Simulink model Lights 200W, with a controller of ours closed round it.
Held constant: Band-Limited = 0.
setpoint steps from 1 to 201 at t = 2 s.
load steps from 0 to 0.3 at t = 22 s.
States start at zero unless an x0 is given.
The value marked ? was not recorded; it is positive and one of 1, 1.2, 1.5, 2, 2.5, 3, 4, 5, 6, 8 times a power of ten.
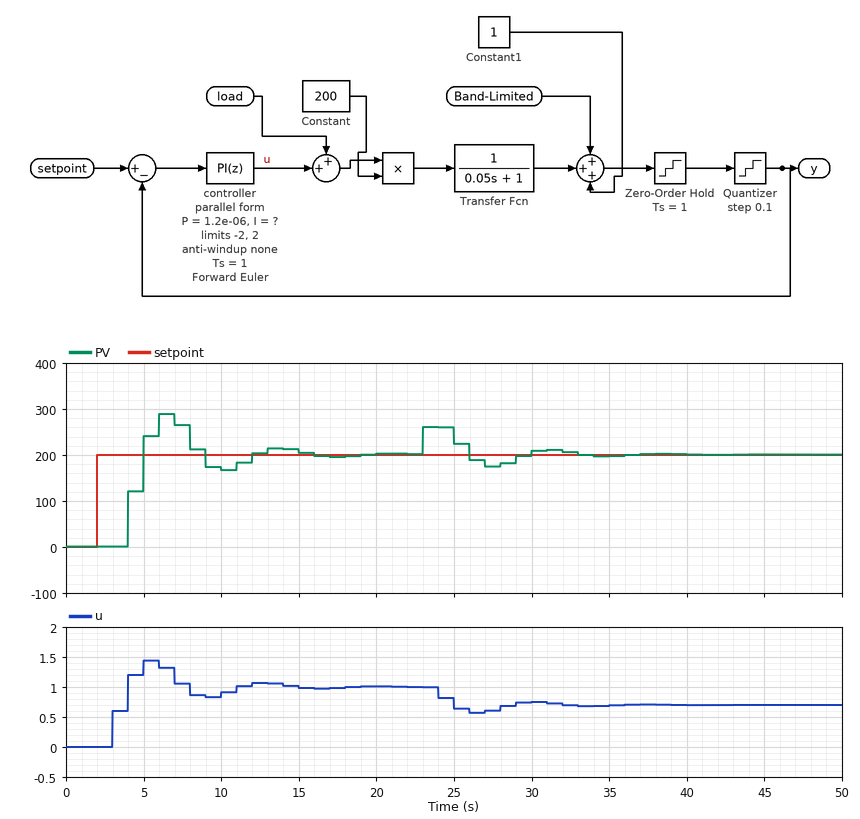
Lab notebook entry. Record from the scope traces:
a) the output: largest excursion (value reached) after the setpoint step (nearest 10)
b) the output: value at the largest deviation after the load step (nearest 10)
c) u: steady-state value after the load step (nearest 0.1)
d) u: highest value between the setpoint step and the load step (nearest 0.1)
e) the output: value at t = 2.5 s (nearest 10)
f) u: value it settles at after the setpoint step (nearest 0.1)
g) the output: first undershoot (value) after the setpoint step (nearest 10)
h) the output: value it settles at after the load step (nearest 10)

290
260
0.7
1.4
0
1.0
170
200
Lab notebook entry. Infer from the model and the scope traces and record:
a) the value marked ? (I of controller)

0.003
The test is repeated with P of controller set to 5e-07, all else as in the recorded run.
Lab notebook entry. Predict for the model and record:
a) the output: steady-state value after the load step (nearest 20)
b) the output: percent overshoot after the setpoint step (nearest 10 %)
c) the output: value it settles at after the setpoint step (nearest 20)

200
40 %
200
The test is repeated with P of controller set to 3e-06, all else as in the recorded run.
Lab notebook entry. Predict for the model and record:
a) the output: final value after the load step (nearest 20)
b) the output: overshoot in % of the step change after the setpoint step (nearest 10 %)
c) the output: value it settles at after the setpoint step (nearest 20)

200
40 %
200
